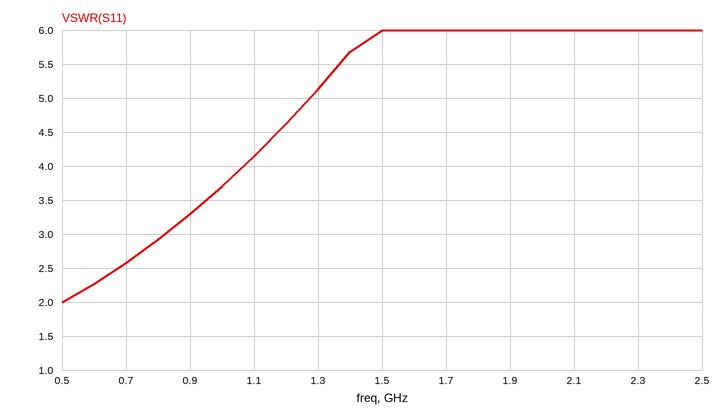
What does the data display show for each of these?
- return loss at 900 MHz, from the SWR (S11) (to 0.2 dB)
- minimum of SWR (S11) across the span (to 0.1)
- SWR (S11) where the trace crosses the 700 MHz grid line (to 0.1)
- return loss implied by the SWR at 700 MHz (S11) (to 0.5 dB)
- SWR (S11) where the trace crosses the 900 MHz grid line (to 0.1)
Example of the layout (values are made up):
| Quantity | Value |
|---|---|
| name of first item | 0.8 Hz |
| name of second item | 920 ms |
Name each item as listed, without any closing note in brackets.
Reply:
| Quantity | Value |
|---|---|
| return loss at 900 MHz, from the SWR (S11) | 5.4 dB |
| minimum of SWR (S11) across the span | 2.0 |
| SWR (S11) where the trace crosses the 700 MHz grid line | 2.6 |
| return loss implied by the SWR at 700 MHz (S11) | 7.0 dB |
| SWR (S11) where the trace crosses the 900 MHz grid line | 3.3 |
